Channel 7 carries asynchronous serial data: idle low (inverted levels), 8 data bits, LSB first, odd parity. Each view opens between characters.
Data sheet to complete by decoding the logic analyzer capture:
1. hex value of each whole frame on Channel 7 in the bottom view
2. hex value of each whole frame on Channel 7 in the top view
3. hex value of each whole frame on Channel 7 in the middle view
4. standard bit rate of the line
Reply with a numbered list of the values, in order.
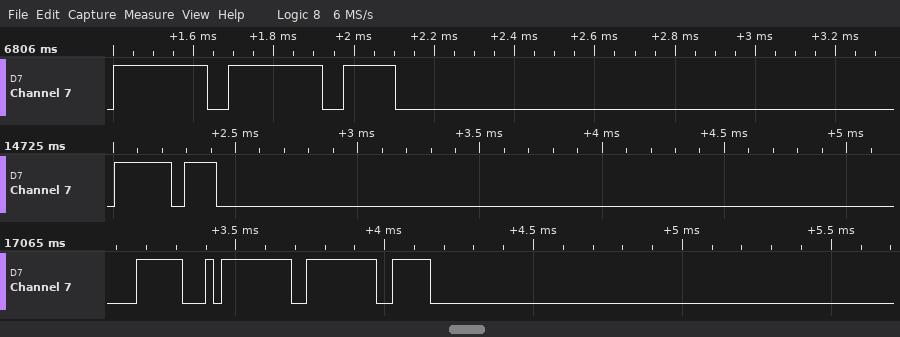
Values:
1. E0, 00, 00, F0
2. 00, 00, F0
3. 00, F0
4. 38400 baud
